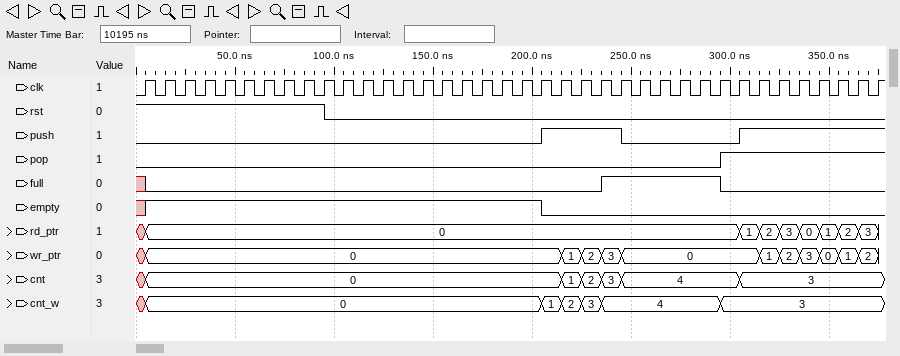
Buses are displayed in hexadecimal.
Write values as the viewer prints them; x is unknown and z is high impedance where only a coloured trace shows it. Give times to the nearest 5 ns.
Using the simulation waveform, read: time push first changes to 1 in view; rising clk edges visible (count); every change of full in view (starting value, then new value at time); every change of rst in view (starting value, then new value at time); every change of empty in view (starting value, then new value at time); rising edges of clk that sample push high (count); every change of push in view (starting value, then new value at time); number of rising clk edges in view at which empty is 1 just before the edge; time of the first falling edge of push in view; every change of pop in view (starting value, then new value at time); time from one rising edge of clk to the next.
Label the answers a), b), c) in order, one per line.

a) 205 ns
b) 38
c) x, 0 at 5 ns, 1 at 235 ns, 0 at 295 ns
d) 1, 0 at 95 ns
e) x, 1 at 5 ns, 0 at 205 ns
f) 11
g) 0, 1 at 205 ns, 0 at 245 ns, 1 at 305 ns
h) 20
i) 245 ns
j) 0, 1 at 295 ns
k) 10 ns
